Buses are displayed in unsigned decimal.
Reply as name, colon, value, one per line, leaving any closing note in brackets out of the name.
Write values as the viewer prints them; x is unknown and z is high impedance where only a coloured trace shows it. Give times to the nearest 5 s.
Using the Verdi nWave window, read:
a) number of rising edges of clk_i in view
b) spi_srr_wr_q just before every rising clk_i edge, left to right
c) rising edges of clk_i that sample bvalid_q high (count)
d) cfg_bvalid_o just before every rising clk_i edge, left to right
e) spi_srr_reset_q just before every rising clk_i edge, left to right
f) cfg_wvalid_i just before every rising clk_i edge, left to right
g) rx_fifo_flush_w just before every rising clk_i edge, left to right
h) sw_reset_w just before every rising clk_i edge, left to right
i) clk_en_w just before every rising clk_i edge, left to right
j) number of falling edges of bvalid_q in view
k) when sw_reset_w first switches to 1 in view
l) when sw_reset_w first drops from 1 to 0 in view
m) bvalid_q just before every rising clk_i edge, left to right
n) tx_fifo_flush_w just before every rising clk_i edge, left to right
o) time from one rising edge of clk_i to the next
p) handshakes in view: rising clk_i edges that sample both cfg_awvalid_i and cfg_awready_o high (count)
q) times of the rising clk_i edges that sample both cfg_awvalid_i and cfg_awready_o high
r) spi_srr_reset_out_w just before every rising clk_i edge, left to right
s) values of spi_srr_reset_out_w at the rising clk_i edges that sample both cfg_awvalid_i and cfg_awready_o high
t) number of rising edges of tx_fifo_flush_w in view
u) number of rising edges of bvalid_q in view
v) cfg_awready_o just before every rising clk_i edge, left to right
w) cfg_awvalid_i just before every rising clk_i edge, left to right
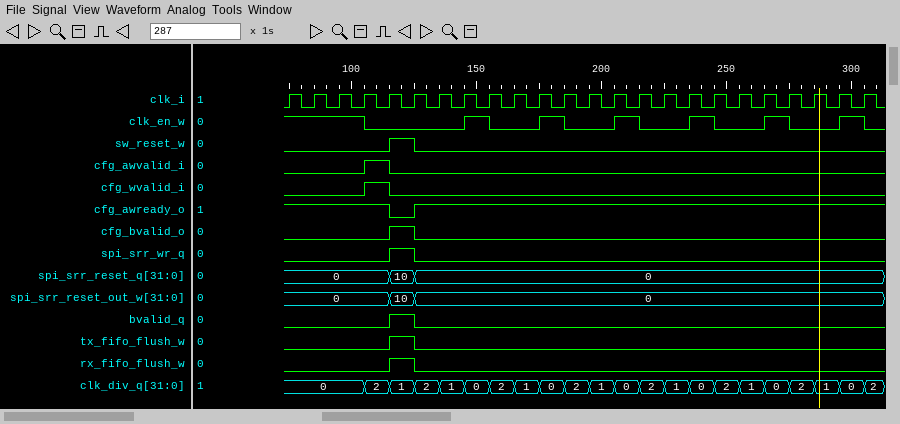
number of rising edges of clk_i in view: 24
spi_srr_wr_q just before every rising clk_i edge, left to right: 0 0 0 0 0 1 0 0 0 0 0 0 0 0 0 0 0 0 0 0 0 0 0 0
rising edges of clk_i that sample bvalid_q high: 1
cfg_bvalid_o just before every rising clk_i edge, left to right: 0 0 0 0 0 1 0 0 0 0 0 0 0 0 0 0 0 0 0 0 0 0 0 0
spi_srr_reset_q just before every rising clk_i edge, left to right: 0, 0, 0, 0, 0, 10, 0, 0, 0, 0, 0, 0, 0, 0, 0, 0, 0, 0, 0, 0, 0, 0, 0, 0
cfg_wvalid_i just before every rising clk_i edge, left to right: 0 0 0 0 1 0 0 0 0 0 0 0 0 0 0 0 0 0 0 0 0 0 0 0
rx_fifo_flush_w just before every rising clk_i edge, left to right: 0 0 0 0 0 1 0 0 0 0 0 0 0 0 0 0 0 0 0 0 0 0 0 0
sw_reset_w just before every rising clk_i edge, left to right: 0 0 0 0 0 1 0 0 0 0 0 0 0 0 0 0 0 0 0 0 0 0 0 0
clk_en_w just before every rising clk_i edge, left to right: 1 1 1 1 0 0 0 0 1 0 0 1 0 0 1 0 0 1 0 0 1 0 0 1
number of falling edges of bvalid_q in view: 1
when sw_reset_w first switches to 1 in view: 115 s
when sw_reset_w first drops from 1 to 0 in view: 125 s
bvalid_q just before every rising clk_i edge, left to right: 0 0 0 0 0 1 0 0 0 0 0 0 0 0 0 0 0 0 0 0 0 0 0 0
tx_fifo_flush_w just before every rising clk_i edge, left to right: 0 0 0 0 0 1 0 0 0 0 0 0 0 0 0 0 0 0 0 0 0 0 0 0
time from one rising edge of clk_i to the next: 10 s
handshakes in view: rising clk_i edges that sample both cfg_awvalid_i and cfg_awready_o high: 1
times of the rising clk_i edges that sample both cfg_awvalid_i and cfg_awready_o high: 115 s
spi_srr_reset_out_w just before every rising clk_i edge, left to right: 0, 0, 0, 0, 0, 10, 0, 0, 0, 0, 0, 0, 0, 0, 0, 0, 0, 0, 0, 0, 0, 0, 0, 0
values of spi_srr_reset_out_w at the rising clk_i edges that sample both cfg_awvalid_i and cfg_awready_o high: 0
number of rising edges of tx_fifo_flush_w in view: 1
number of rising edges of bvalid_q in view: 1
cfg_awready_o just before every rising clk_i edge, left to right: 1 1 1 1 1 0 1 1 1 1 1 1 1 1 1 1 1 1 1 1 1 1 1 1
cfg_awvalid_i just before every rising clk_i edge, left to right: 0 0 0 0 1 0 0 0 0 0 0 0 0 0 0 0 0 0 0 0 0 0 0 0
